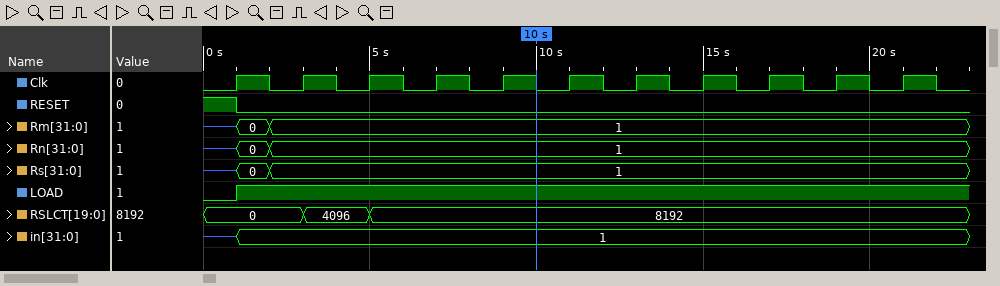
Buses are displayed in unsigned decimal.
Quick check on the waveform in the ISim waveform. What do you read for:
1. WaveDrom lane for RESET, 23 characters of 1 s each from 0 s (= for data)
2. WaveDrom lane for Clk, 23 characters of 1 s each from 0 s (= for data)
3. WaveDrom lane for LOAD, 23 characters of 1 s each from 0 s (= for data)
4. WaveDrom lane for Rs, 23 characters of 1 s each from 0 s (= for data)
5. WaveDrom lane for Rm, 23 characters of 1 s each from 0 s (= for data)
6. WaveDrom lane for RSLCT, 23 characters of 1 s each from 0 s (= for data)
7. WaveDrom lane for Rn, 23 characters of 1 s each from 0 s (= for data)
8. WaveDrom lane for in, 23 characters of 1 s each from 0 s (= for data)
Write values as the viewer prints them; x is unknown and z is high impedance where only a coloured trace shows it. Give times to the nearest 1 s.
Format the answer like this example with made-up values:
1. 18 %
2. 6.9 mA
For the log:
1. {name: 'RESET', wave: '10.....................'}
2. {name: 'Clk', wave: '01010101010101010101010'}
3. {name: 'LOAD', wave: '01.....................'}
4. {name: 'Rs', wave: 'z==....................', data: '0 1'}
5. {name: 'Rm', wave: 'z==....................', data: '0 1'}
6. {name: 'RSLCT', wave: '=..=.=.................', data: '0 4096 8192'}
7. {name: 'Rn', wave: 'z==....................', data: '0 1'}
8. {name: 'in', wave: 'z=.....................', data: '1'}
